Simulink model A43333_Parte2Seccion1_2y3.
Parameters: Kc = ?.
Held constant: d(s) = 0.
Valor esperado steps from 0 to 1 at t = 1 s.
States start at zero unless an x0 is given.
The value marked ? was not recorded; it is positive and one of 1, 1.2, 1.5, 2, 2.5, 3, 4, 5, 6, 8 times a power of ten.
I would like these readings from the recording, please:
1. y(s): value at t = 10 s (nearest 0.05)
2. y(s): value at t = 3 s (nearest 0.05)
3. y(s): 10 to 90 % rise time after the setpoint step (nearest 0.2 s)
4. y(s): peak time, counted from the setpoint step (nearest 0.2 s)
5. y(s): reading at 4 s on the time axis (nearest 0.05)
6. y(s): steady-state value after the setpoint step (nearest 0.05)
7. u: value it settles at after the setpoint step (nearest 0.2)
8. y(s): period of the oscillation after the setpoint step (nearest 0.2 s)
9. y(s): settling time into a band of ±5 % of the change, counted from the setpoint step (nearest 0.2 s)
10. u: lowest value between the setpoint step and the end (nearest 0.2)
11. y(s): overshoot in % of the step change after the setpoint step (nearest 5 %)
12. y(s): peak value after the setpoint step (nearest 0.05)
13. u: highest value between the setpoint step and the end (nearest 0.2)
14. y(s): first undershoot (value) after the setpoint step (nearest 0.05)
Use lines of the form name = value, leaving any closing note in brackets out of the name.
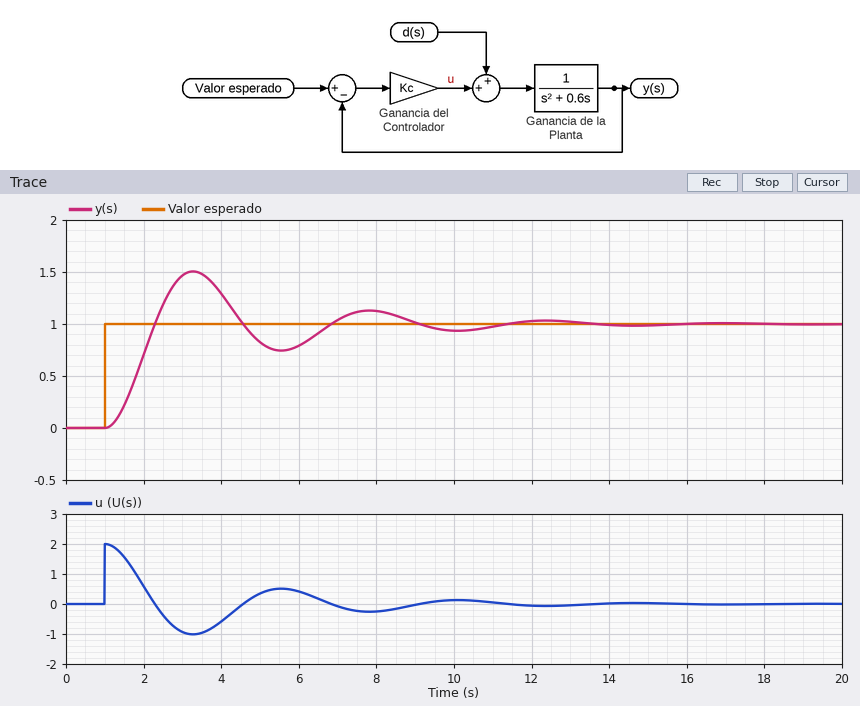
y(s): value at t = 10 s = 0.95
y(s): value at t = 3 s = 1.45
y(s): 10 to 90 % rise time after the setpoint step = 0.8 s
y(s): peak time, counted from the setpoint step = 2.2 s
y(s): reading at 4 s on the time axis = 1.30
y(s): steady-state value after the setpoint step = 1.00
u: value it settles at after the setpoint step = 0.0
y(s): period of the oscillation after the setpoint step = 4.6 s
y(s): settling time into a band of ±5 % of the change, counted from the setpoint step = 9.6 s
u: lowest value between the setpoint step and the end = -1.0
y(s): overshoot in % of the step change after the setpoint step = 50 %
y(s): peak value after the setpoint step = 1.50
u: highest value between the setpoint step and the end = 2.0
y(s): first undershoot (value) after the setpoint step = 0.75
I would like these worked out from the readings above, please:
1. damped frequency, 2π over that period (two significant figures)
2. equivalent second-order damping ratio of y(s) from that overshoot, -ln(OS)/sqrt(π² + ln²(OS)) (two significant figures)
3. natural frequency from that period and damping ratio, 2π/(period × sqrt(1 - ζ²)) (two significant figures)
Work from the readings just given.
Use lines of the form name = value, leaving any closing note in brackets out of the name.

damped frequency, 2π over that period = 1.4 rad/s
equivalent second-order damping ratio of y(s) from that overshoot, -ln(OS)/sqrt(π² + ln²(OS)) = 0.22
natural frequency from that period and damping ratio, 2π/(period × sqrt(1 - ζ²)) = 1.4 rad/s
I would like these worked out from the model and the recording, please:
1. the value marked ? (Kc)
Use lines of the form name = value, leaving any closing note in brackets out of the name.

the value marked ? = 2
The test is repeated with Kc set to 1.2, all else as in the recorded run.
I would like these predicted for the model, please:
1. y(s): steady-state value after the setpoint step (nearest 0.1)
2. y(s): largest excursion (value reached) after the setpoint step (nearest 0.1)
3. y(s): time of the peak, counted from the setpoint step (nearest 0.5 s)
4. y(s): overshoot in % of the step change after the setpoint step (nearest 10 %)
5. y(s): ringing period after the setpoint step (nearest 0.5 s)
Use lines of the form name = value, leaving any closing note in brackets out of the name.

y(s): steady-state value after the setpoint step = 1.0
y(s): largest excursion (value reached) after the setpoint step = 1.4
y(s): time of the peak, counted from the setpoint step = 3.0 s
y(s): overshoot in % of the step change after the setpoint step = 40 %
y(s): ringing period after the setpoint step = 6.0 s
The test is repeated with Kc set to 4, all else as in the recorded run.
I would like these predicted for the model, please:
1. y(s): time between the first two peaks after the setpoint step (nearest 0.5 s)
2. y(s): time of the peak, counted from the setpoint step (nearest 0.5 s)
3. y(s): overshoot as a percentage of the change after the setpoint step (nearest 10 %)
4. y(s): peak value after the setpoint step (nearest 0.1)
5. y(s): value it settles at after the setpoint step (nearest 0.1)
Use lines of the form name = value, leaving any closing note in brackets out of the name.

y(s): time between the first two peaks after the setpoint step = 3.0 s
y(s): time of the peak, counted from the setpoint step = 1.5 s
y(s): overshoot as a percentage of the change after the setpoint step = 60 %
y(s): peak value after the setpoint step = 1.6
y(s): value it settles at after the setpoint step = 1.0
